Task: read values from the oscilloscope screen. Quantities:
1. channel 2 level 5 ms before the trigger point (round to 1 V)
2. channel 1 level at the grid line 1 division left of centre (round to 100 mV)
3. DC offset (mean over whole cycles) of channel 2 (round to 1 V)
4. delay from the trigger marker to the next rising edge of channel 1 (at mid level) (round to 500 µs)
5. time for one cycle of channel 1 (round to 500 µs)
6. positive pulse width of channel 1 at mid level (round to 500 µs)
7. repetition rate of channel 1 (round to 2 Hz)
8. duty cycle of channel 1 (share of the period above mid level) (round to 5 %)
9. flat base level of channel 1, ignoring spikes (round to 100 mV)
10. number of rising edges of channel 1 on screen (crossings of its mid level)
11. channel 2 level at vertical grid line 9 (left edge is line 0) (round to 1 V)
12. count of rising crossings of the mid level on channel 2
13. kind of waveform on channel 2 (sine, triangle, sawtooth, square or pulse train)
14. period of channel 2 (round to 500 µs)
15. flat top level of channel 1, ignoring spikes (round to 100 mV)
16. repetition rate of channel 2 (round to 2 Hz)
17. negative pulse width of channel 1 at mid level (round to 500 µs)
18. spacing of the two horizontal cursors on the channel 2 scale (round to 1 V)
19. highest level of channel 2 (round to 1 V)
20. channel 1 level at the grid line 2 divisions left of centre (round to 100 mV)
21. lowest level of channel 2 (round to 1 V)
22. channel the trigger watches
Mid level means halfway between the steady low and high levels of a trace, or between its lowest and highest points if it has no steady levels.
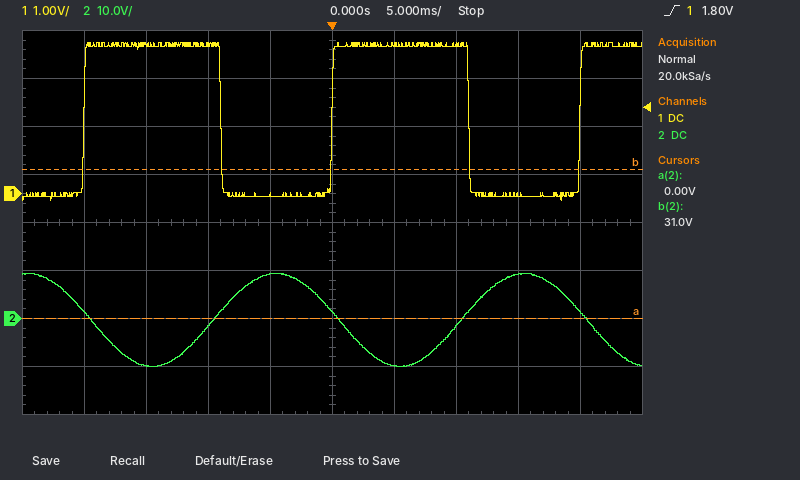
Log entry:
9 V
0.0 V
0 V
20.0 ms
20.0 ms
11.0 ms
50 Hz
55 %
-100 mV
3
1 V
2
sine
20.0 ms
3.1 V
50 Hz
9.0 ms
31 V
9 V
3.1 V
-10 V
channel 1
